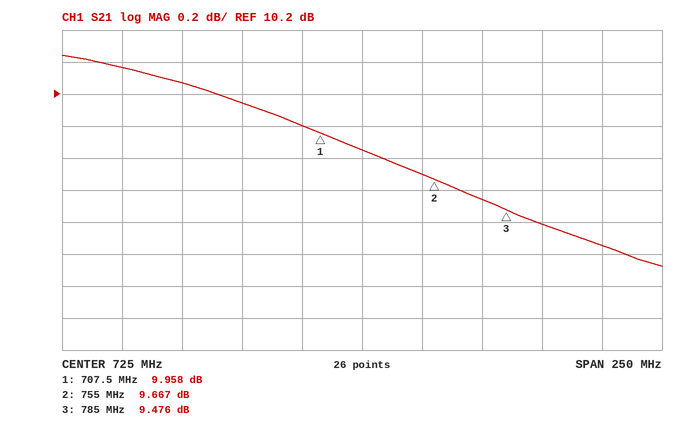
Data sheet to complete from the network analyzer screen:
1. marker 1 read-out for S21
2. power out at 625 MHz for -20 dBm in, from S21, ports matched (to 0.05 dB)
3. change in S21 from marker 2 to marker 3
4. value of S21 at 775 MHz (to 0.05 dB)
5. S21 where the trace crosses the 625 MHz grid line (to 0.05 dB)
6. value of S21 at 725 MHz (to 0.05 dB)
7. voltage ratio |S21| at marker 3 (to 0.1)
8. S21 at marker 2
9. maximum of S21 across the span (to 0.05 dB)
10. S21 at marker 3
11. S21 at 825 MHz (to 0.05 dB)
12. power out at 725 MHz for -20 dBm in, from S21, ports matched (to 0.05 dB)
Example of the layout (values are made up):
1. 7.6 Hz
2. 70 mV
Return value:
1. 9.958 dB
2. -9.65 dBm
3. -0.191 dB
4. 9.55 dB
5. 10.35 dB
6. 9.85 dB
7. 3.0
8. 9.667 dB
9. 10.45 dB
10. 9.476 dB
11. 9.25 dB
12. -10.15 dBm
